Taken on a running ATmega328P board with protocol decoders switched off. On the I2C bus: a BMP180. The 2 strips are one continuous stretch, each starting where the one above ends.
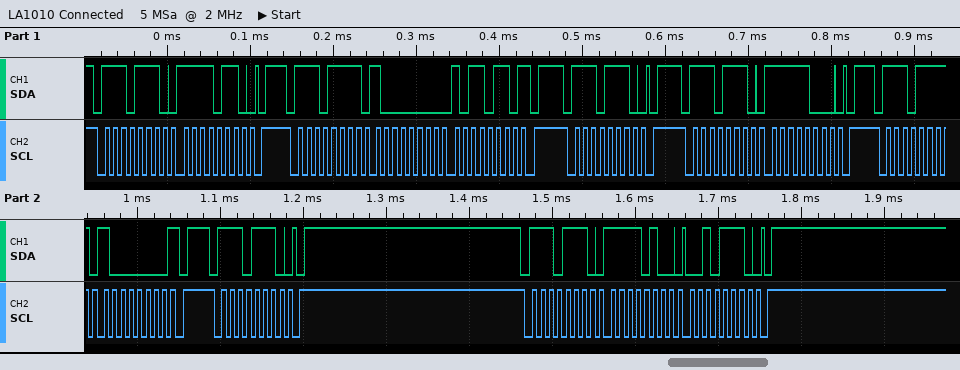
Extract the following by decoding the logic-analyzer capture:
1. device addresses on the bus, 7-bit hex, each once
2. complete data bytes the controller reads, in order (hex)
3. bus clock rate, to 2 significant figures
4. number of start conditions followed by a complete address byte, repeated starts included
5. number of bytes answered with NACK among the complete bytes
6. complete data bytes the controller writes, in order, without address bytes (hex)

0x77
80 B6 80
100 kHz
7
2
F6 F8 F4 2E
